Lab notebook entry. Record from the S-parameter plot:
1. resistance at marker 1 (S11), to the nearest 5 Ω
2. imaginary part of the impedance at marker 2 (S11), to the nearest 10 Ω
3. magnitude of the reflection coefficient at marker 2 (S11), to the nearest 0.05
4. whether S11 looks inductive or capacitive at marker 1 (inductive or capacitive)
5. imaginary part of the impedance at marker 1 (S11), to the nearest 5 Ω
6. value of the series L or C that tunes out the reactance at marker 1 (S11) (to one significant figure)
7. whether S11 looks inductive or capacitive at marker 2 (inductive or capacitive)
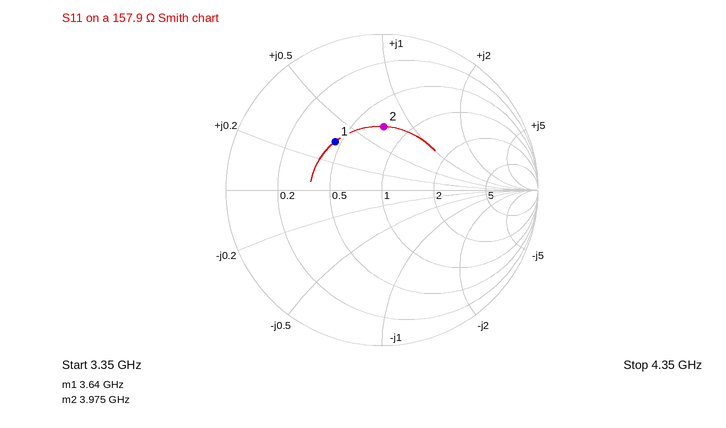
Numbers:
70 Ω
+110 Ω
0.40
inductive
+55 Ω
800 fF
inductive
